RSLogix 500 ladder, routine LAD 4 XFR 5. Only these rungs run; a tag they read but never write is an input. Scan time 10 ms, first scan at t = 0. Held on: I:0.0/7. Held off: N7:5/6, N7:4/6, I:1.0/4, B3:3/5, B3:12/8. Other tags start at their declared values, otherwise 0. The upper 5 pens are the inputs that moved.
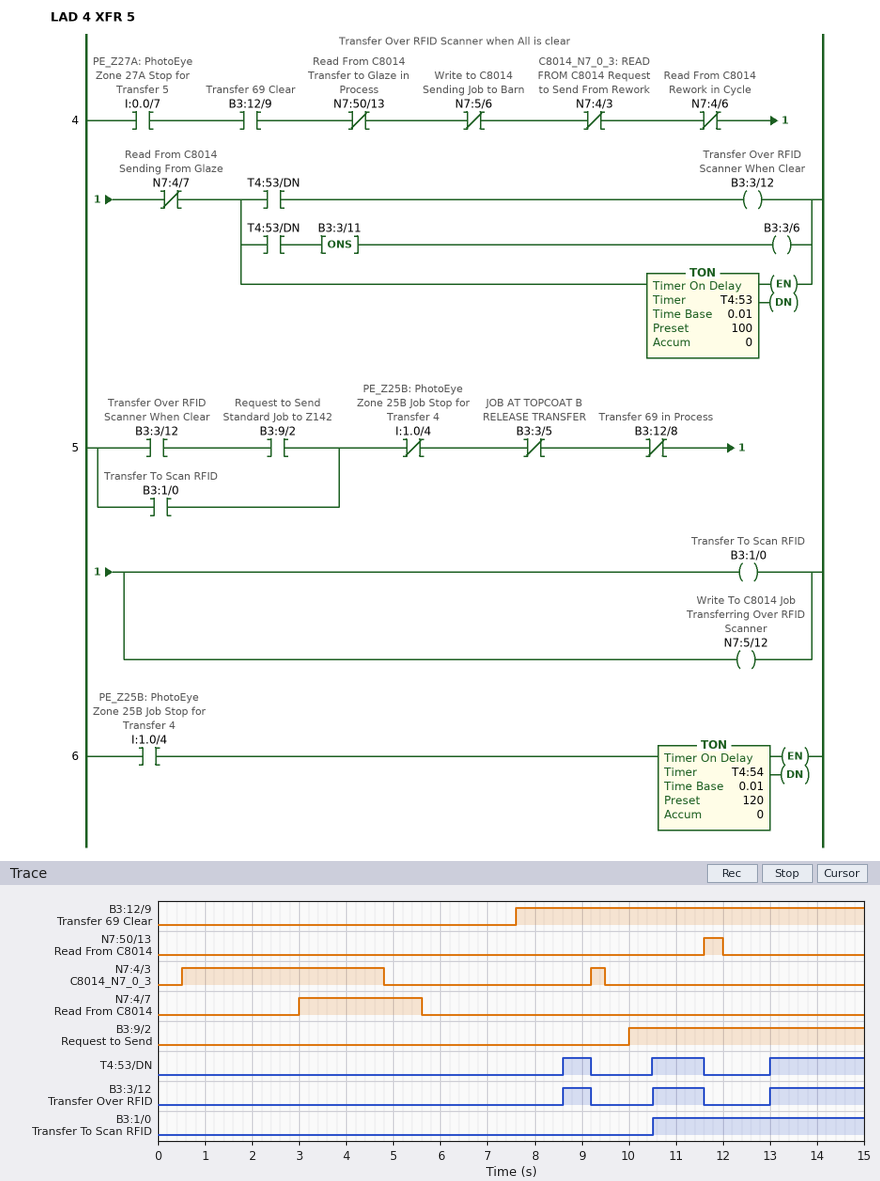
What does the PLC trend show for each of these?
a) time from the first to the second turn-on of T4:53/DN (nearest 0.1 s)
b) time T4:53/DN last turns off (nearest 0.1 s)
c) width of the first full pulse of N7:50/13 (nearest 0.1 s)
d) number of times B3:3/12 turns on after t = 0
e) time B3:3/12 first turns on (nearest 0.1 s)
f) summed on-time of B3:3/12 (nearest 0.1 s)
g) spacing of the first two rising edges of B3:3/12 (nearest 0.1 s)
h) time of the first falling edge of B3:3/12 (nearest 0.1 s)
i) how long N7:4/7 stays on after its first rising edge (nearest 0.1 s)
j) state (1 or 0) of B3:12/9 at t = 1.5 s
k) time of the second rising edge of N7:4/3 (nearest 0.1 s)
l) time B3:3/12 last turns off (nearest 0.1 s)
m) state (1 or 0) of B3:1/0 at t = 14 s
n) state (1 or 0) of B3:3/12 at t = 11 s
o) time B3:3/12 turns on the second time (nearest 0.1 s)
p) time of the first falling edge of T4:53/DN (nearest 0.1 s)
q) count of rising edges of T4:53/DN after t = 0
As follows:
1.9 s
11.6 s
0.4 s
3
8.6 s
3.7 s
1.9 s
9.2 s
2.6 s
0
9.2 s
11.6 s
1
1
10.5 s
9.2 s
3
